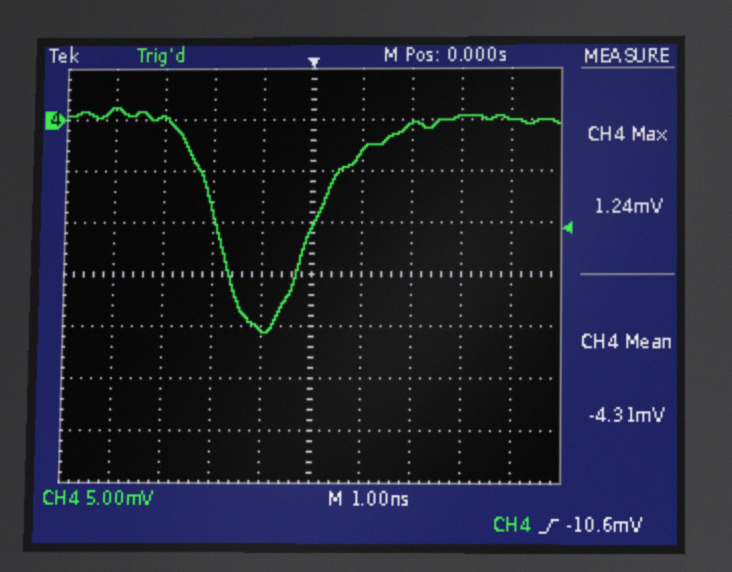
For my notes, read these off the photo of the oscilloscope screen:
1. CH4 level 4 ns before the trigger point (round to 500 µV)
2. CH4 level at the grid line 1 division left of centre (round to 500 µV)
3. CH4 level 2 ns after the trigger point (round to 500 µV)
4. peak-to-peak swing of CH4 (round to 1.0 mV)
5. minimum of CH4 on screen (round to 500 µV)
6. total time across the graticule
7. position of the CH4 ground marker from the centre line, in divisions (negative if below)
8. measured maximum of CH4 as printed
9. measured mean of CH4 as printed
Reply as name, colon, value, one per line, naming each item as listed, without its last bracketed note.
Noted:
CH4 level 4 ns before the trigger point: 1.0 mV
CH4 level at the grid line 1 division left of centre: -20.5 mV
CH4 level 2 ns after the trigger point: -500 µV
peak-to-peak swing of CH4: 22.0 mV
minimum of CH4 on screen: -20.5 mV
total time across the graticule: 10 ns
position of the CH4 ground marker from the centre line, in divisions: +3.0 div
measured maximum of CH4 as printed: 1.24 mV
measured mean of CH4 as printed: -4.31 mV
